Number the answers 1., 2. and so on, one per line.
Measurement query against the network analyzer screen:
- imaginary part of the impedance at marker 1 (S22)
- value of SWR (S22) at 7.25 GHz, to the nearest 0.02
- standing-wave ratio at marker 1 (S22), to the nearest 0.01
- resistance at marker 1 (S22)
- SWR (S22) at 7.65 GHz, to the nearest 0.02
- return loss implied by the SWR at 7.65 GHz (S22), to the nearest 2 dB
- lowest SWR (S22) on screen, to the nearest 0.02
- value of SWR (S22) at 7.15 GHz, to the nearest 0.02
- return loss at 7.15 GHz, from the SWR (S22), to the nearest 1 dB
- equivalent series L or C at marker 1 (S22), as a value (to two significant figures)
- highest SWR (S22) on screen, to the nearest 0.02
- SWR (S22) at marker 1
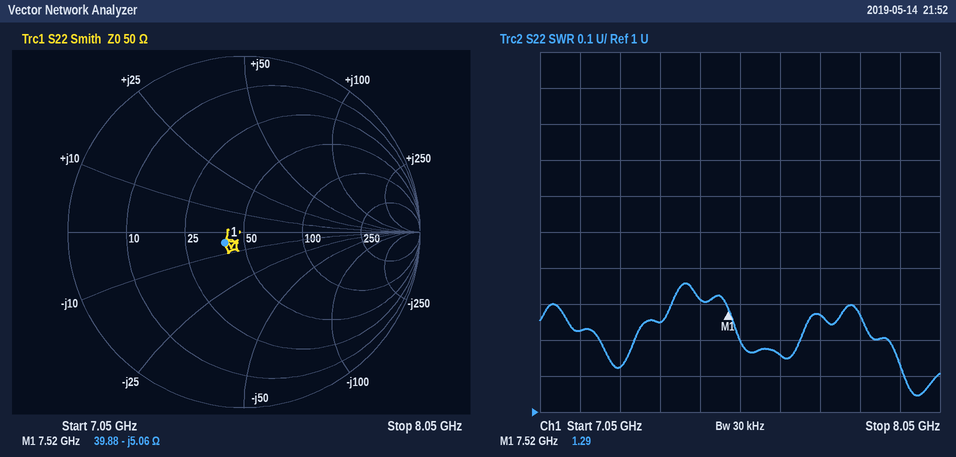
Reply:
1. -5.06 Ω
2. 1.12
3. 1.29
4. 39.88 Ω
5. 1.16
6. 22 dB
7. 1.04
8. 1.22
9. 20 dB
10. 4.2 pF
11. 1.36
12. 1.29
